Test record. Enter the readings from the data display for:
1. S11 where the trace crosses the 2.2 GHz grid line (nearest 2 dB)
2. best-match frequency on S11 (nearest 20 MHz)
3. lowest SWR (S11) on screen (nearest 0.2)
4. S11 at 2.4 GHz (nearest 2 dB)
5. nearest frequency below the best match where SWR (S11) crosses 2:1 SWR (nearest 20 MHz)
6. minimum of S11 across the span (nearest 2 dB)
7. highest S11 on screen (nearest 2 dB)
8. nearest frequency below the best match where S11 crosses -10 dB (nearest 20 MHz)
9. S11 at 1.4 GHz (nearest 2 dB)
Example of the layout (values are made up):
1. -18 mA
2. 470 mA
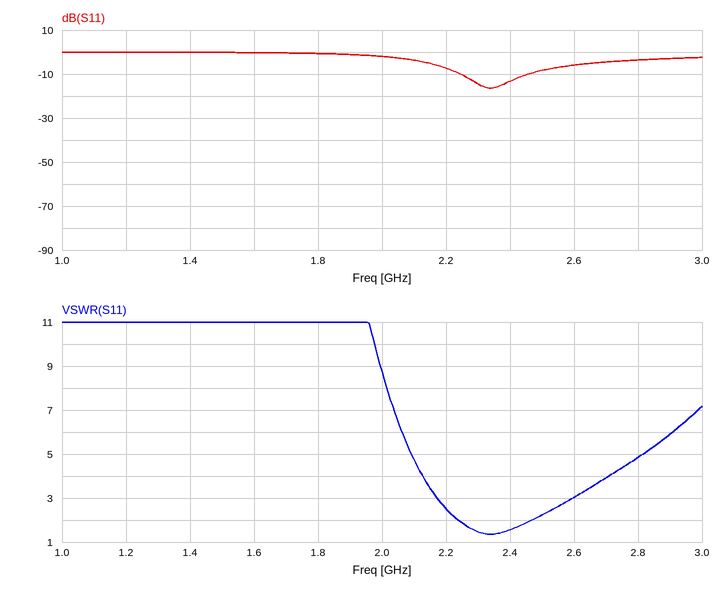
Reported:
1. -8 dB
2. 2.34 GHz
3. 1.4
4. -14 dB
5. 2.24 GHz
6. -16 dB
7. 0 dB
8. 2.24 GHz
9. 0 dB
